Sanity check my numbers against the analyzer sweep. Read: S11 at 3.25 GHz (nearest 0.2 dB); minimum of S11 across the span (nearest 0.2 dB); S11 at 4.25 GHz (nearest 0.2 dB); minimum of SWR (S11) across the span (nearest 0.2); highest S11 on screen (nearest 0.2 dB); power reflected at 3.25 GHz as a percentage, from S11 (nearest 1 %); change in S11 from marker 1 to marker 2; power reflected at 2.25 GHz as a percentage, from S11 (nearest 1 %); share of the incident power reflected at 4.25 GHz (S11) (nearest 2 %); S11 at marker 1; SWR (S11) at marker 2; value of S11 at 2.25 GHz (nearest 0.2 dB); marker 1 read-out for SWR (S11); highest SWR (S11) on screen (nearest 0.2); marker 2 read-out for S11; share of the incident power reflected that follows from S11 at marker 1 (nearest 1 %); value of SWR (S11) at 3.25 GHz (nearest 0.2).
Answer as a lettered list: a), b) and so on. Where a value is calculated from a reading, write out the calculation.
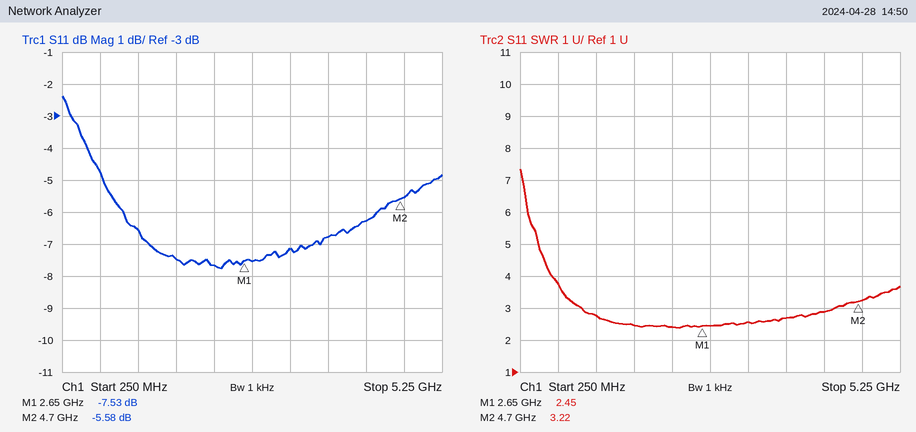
a) -7.2 dB
b) -7.8 dB
c) -6.2 dB
d) 2.4
e) -2.4 dB
f) 10^(-7.2/10) ≈ 19 %
g) -5.58 − (-7.53) = 1.95 dB
h) 10^(-7.6/10) ≈ 17 %
i) 10^(-6.2/10) ≈ 24 %
j) -7.53 dB
k) 3.22
l) -7.6 dB
m) 2.45
n) 7.4
o) -5.58 dB
p) 10^(-7.53/10) ≈ 18 %
q) 2.6
